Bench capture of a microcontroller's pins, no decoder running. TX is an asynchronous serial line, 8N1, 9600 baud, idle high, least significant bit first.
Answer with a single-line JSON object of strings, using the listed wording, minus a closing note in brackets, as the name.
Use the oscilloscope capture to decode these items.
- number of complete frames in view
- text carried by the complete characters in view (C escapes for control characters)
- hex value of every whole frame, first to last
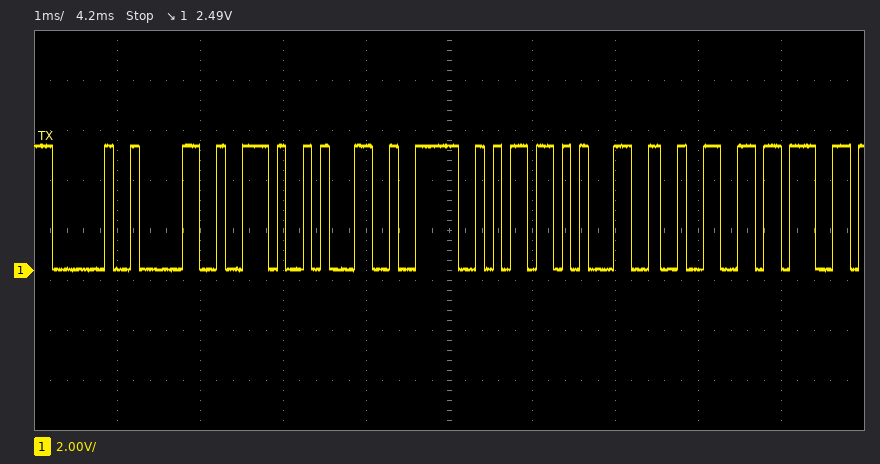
{"number of complete frames in view": "9", "text carried by the complete characters in view": "\" 0.1>m12;\"", "hex value of every whole frame, first to last": "0x20 0x30 0x2E 0x31 0x3E 0x6D 0x31 0x32 0x3B"}
